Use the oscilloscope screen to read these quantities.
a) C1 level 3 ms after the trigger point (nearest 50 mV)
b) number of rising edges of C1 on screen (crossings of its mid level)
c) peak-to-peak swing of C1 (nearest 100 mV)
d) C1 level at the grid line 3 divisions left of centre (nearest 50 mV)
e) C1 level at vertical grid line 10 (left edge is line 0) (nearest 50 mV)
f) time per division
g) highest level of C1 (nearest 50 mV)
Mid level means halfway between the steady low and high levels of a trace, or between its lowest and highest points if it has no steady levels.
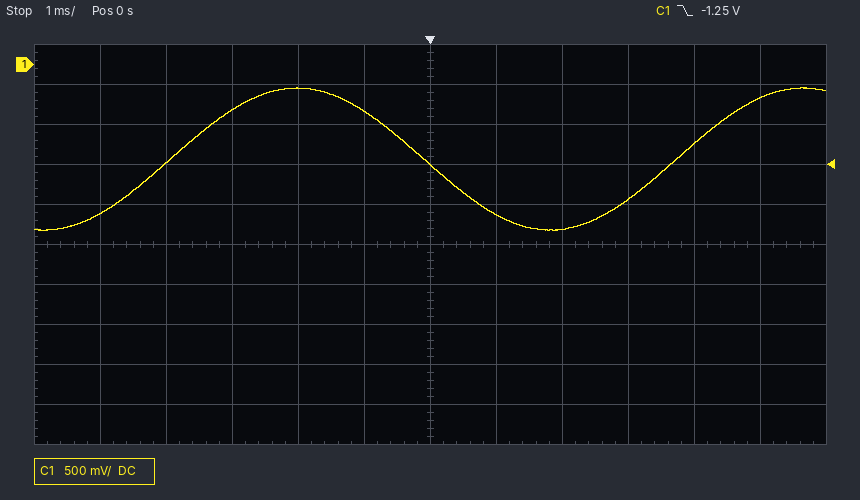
-1.70 V
2
1.80 V
-550 mV
-1.00 V
1 ms
-300 mV
